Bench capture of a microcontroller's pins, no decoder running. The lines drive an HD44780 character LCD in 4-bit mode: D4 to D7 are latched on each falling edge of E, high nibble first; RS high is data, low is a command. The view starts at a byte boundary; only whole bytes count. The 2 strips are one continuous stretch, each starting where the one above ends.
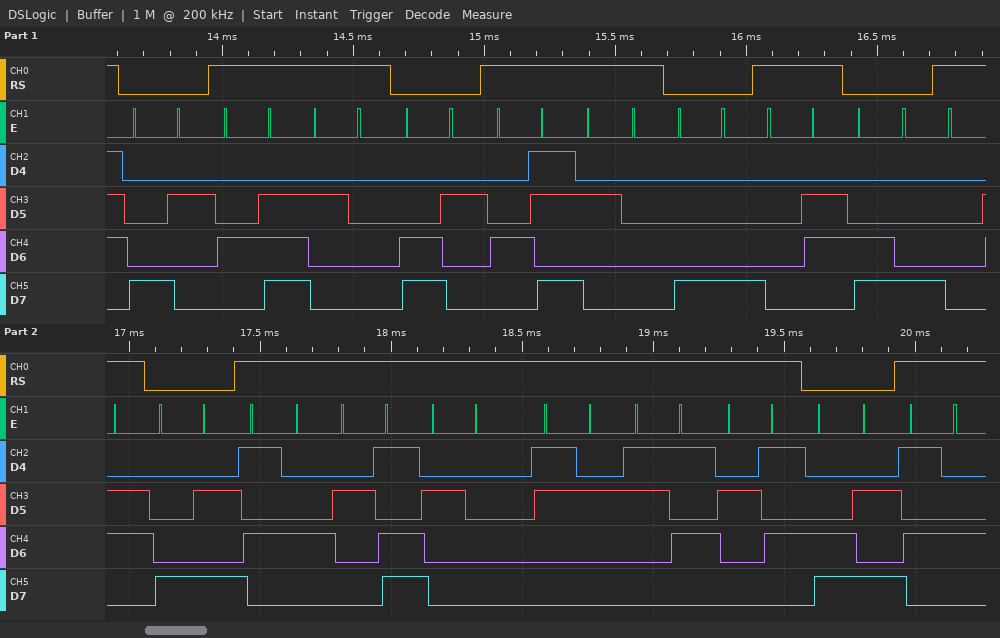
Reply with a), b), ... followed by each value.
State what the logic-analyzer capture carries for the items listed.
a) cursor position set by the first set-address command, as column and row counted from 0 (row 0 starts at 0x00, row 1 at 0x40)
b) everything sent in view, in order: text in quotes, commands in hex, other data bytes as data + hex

a) column 2, row 0
b) 0x82 "N " 0xC2 "K " 0x88 data 06 0xC8 data 06 0x8A "T- 25%" 0xCA "T"
